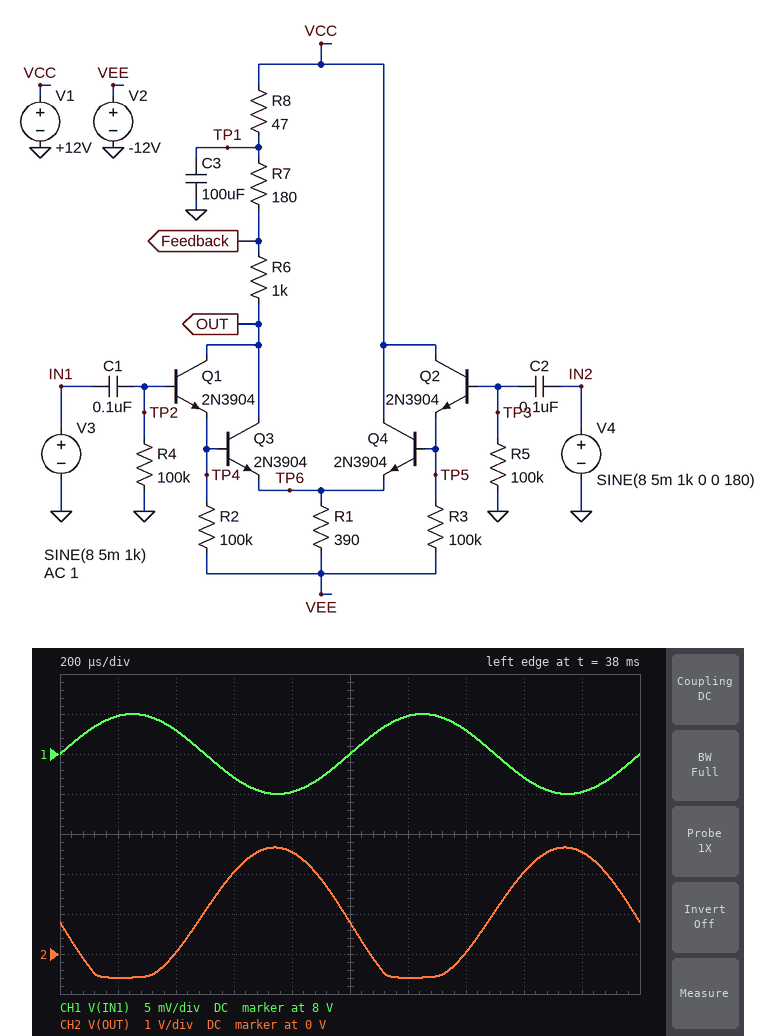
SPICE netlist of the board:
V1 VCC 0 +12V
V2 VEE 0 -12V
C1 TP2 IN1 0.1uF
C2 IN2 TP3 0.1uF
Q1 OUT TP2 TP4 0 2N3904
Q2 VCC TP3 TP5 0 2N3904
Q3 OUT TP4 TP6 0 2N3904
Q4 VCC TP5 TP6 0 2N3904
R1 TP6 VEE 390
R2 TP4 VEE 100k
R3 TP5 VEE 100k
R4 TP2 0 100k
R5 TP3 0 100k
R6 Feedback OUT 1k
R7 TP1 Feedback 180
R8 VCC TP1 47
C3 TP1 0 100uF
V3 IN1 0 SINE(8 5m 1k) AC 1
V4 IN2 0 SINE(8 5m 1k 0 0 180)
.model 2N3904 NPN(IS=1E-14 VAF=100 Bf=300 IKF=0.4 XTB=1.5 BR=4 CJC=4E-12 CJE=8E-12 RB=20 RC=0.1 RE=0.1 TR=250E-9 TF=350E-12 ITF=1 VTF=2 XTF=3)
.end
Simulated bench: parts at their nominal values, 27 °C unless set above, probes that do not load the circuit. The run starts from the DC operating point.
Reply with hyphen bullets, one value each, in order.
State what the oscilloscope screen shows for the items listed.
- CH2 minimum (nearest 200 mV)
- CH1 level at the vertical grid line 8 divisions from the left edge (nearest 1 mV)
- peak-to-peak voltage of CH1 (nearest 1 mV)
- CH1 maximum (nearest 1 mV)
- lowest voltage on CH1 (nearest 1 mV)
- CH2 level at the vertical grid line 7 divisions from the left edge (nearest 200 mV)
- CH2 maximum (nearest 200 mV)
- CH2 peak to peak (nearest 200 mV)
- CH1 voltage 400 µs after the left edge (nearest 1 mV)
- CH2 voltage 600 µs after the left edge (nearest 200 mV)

- -600 mV
- 7.997 V
- 10 mV
- 8.005 V
- 7.995 V
- 0 V
- 2.6 V
- 3.2 V
- 8.003 V
- 2.0 V
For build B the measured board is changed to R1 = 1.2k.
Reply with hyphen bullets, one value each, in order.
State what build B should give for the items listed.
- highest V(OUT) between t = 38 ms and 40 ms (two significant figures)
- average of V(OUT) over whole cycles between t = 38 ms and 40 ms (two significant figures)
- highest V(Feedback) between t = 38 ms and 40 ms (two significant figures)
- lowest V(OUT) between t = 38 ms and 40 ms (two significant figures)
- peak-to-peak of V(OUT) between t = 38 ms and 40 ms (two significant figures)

- 7.6 V
- 6.8 V
- 11 V
- 5.9 V
- 1.7 V
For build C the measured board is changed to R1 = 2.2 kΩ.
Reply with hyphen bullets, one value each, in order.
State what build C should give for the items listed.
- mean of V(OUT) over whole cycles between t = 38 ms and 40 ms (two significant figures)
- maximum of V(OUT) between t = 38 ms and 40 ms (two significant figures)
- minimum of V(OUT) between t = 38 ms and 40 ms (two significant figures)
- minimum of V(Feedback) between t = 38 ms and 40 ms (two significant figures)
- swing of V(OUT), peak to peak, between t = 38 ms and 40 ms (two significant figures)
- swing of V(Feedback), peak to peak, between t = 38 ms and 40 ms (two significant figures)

- 9.0 V
- 9.5 V
- 8.5 V
- 11 V
- 990 mV
- 150 mV
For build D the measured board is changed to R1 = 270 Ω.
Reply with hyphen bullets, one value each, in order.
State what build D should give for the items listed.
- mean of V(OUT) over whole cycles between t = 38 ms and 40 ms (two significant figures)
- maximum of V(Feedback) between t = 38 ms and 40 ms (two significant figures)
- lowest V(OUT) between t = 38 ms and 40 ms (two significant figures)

- 820 mV
- 10 V
- -640 mV
